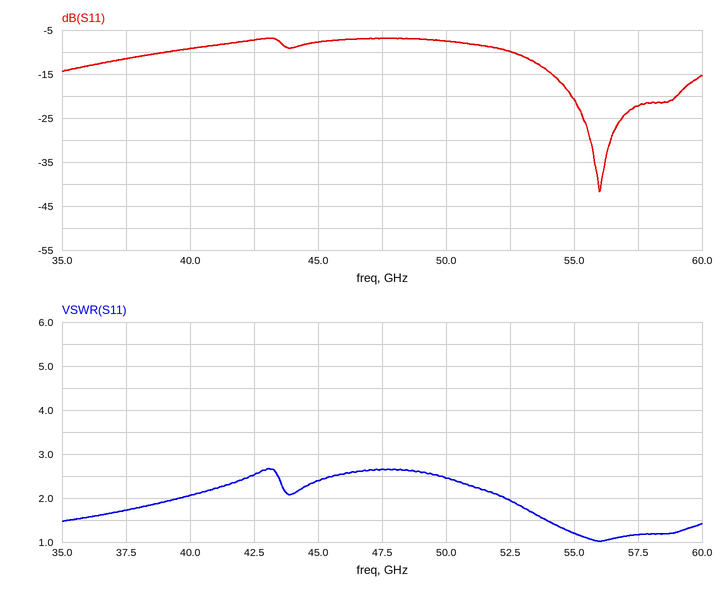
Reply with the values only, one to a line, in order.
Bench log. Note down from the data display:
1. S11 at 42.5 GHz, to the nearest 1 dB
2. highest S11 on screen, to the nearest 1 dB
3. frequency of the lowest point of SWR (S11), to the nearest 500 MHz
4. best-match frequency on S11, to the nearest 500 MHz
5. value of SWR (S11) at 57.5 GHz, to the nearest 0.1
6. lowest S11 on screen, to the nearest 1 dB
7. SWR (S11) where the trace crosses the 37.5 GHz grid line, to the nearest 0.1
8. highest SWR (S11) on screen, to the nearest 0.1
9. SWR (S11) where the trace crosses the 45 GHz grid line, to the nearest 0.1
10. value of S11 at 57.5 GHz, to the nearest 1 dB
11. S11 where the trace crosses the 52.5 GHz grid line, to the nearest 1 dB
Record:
-7 dB
-7 dB
56.0 GHz
56.0 GHz
1.2
-42 dB
1.7
2.7
2.4
-22 dB
-10 dB
